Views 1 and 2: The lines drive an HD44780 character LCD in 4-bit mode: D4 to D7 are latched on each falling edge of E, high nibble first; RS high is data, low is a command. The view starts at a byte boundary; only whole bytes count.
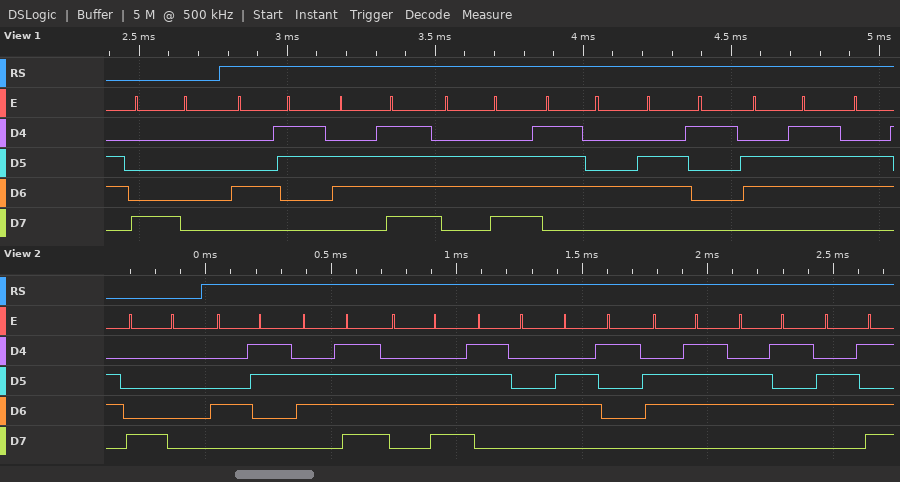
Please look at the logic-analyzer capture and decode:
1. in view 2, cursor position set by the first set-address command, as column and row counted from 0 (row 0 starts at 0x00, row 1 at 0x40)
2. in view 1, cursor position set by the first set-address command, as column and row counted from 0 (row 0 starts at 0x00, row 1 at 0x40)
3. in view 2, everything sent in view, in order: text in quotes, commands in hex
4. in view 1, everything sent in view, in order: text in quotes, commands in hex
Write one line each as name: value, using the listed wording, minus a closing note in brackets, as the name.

in view 2, cursor position set by the first set-address command, as column and row counted from 0: column 0, row 0
in view 1, cursor position set by the first set-address command, as column and row counted from 0: column 0, row 0
in view 2, everything sent in view, in order: text in quotes, commands in hex: 0x80 "Contagem"
in view 1, everything sent in view, in order: text in quotes, commands in hex: 0x80 "Contag"
